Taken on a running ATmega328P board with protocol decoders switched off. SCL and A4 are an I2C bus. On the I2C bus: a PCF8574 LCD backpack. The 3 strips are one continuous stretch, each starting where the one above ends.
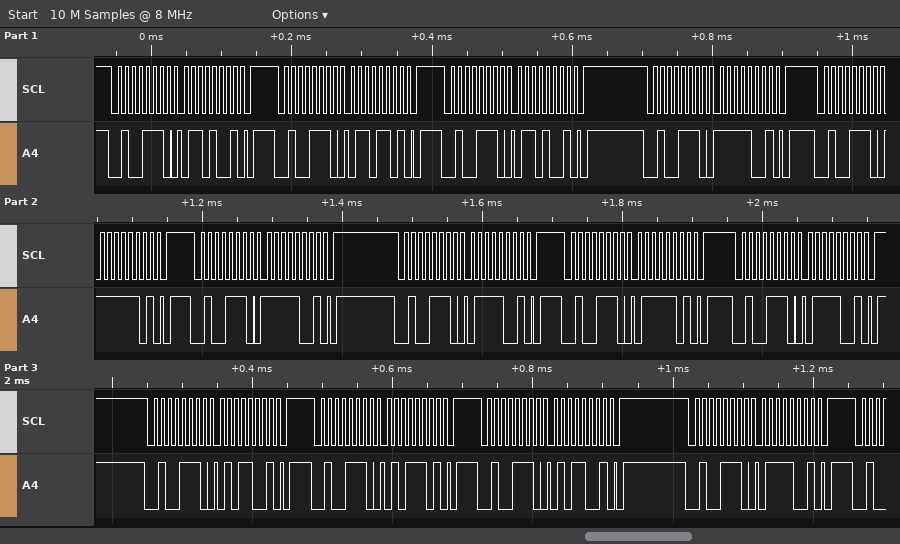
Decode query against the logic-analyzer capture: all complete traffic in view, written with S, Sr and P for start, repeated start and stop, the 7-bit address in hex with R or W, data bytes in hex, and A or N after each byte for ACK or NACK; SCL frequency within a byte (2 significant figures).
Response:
S 27W A 69 A P S 27W A 6D A P S 27W A 69 A P S 27W A F9 A P S 27W A FD A P S 27W A F9 A P S 27W A 79 A P S 27W A 7D A P S 27W A 79 A P S 27W A 59 A P S 27W A 5D A P S 27W A 59 A P S 27W A 79 A P
100 kHz
